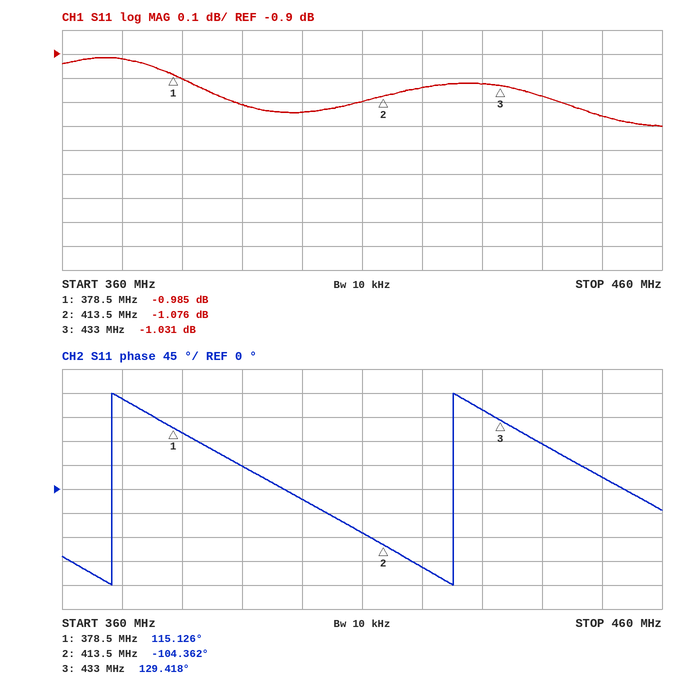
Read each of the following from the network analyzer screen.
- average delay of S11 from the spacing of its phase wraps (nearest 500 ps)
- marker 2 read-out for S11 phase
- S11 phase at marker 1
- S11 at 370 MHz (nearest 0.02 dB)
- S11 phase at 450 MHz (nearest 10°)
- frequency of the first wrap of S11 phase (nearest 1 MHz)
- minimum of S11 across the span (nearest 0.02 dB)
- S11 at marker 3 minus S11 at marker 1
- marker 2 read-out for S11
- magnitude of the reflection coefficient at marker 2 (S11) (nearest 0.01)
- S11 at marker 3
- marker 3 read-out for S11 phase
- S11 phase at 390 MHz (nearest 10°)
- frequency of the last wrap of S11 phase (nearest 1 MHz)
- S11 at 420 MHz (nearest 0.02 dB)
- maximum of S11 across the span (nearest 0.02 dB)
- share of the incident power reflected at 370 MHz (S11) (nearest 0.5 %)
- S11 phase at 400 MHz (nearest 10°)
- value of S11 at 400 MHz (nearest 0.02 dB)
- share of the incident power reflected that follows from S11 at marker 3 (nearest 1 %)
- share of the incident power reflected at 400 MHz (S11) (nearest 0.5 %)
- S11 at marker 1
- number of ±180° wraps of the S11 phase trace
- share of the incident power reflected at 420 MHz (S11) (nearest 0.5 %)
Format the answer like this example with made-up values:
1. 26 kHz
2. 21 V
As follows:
1. 17.5 ns
2. -104.362°
3. 115.126°
4. -0.92 dB
5. 20°
6. 368 MHz
7. -1.20 dB
8. -0.046 dB
9. -1.076 dB
10. 0.88
11. -1.031 dB
12. 129.418°
13. 40°
14. 425 MHz
15. -1.04 dB
16. -0.92 dB
17. 81.0 %
18. -20°
19. -1.14 dB
20. 79 %
21. 77.0 %
22. -0.985 dB
23. 2
24. 78.5 %
